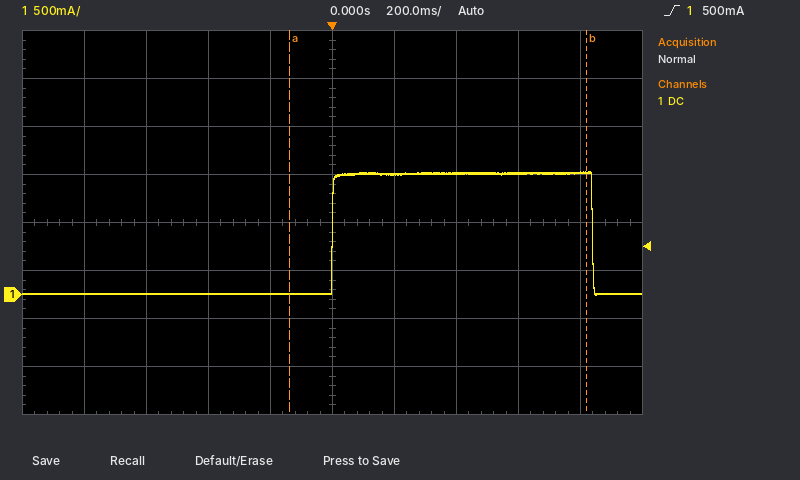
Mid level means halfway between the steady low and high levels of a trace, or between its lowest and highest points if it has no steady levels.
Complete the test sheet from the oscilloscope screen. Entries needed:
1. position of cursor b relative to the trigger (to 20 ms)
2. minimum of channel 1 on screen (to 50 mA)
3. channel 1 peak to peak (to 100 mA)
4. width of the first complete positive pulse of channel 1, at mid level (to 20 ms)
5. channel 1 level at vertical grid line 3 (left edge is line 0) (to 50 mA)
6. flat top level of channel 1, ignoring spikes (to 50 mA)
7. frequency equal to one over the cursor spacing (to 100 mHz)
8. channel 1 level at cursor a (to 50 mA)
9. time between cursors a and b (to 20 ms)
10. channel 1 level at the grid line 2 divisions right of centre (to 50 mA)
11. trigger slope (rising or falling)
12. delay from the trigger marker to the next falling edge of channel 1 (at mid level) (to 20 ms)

+820 ms
0 mA
1.30 A
840 ms
0 mA
1.25 A
1.0 Hz
0 mA
960 ms
1.25 A
rising
840 ms
